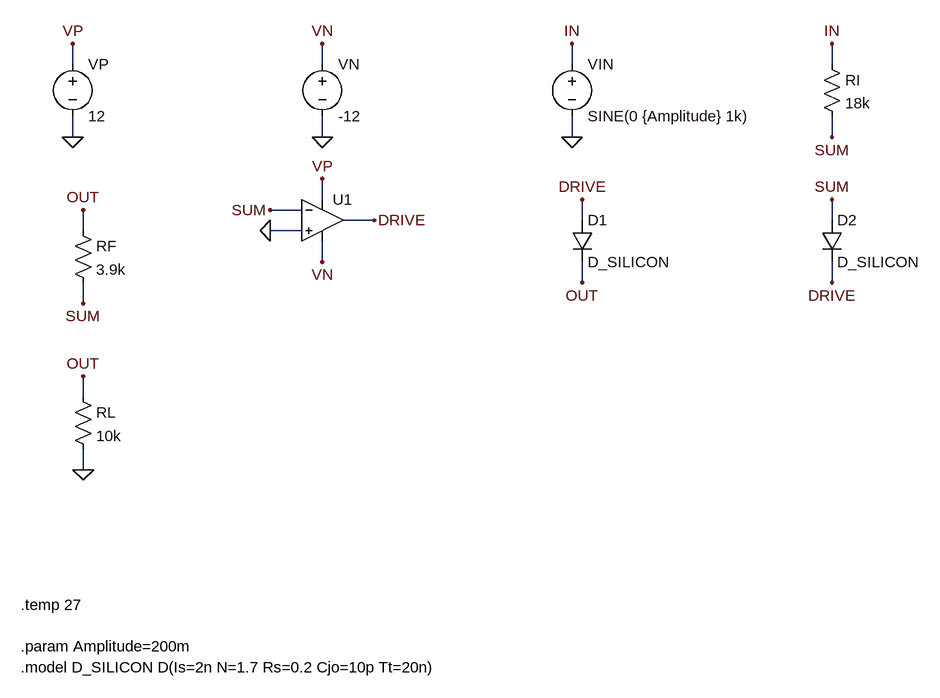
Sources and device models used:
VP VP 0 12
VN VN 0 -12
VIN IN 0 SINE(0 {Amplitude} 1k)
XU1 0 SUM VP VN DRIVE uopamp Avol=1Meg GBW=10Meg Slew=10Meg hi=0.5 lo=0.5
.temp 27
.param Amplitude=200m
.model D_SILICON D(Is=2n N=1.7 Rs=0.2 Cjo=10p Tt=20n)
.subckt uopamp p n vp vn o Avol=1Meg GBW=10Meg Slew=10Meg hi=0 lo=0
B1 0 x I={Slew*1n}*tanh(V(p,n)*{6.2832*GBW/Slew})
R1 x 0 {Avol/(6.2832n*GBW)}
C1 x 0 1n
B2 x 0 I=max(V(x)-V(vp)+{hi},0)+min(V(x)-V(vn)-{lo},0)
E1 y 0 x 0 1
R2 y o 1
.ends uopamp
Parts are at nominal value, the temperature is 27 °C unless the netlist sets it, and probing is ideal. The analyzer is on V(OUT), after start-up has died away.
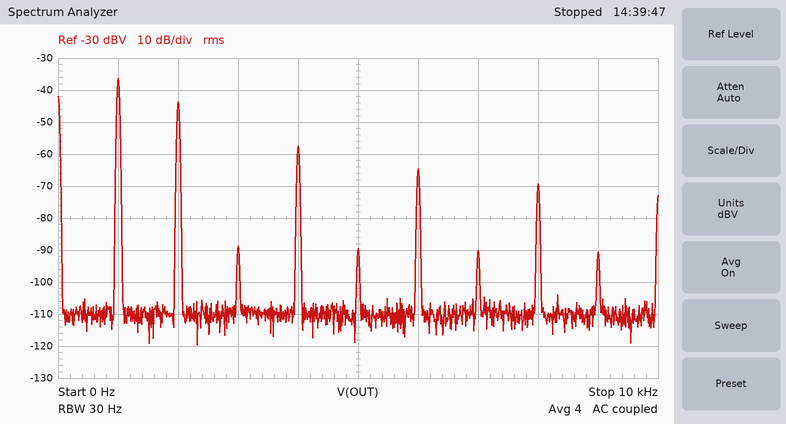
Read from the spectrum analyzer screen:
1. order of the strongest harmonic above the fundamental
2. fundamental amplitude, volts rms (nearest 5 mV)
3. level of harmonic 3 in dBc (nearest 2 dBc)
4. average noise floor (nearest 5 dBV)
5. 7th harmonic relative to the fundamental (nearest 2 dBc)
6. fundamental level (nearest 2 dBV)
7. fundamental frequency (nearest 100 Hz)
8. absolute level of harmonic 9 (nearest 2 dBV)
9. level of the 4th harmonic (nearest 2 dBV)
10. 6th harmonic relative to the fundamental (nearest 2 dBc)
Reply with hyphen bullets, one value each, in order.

- 2
- 15 mV
- -52 dBc
- -110 dBV
- -54 dBc
- -36 dBV
- 1.0 kHz
- -90 dBV
- -58 dBV
- -28 dBc
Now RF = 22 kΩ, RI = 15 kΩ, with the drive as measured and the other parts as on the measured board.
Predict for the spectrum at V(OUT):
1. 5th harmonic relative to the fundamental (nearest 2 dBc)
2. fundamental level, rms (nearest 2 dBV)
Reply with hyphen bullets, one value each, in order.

- -56 dBc
- -20 dBV
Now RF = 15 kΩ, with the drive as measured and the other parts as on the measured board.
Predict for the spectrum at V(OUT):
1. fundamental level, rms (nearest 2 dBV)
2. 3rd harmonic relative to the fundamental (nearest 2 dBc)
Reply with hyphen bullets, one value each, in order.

- -24 dBV
- -54 dBc
